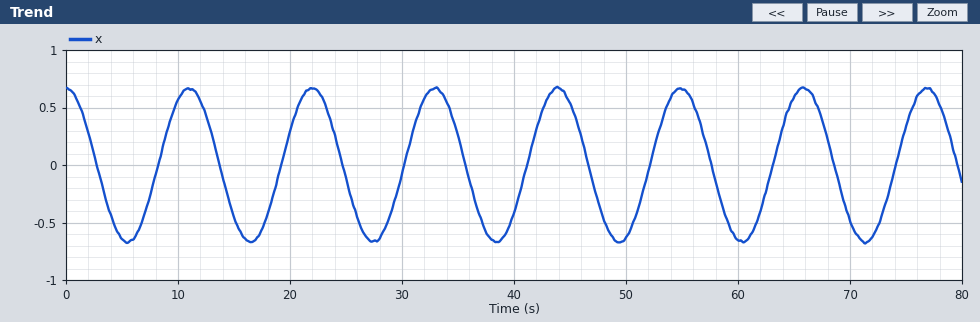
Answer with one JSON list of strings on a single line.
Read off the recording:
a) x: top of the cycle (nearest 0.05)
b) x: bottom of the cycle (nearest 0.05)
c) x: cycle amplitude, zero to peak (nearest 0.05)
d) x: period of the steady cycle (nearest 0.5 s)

["0.65", "-0.65", "0.65", "11.0 s"]
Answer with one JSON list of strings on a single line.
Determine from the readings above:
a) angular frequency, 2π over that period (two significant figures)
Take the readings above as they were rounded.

["0.57 rad/s"]
